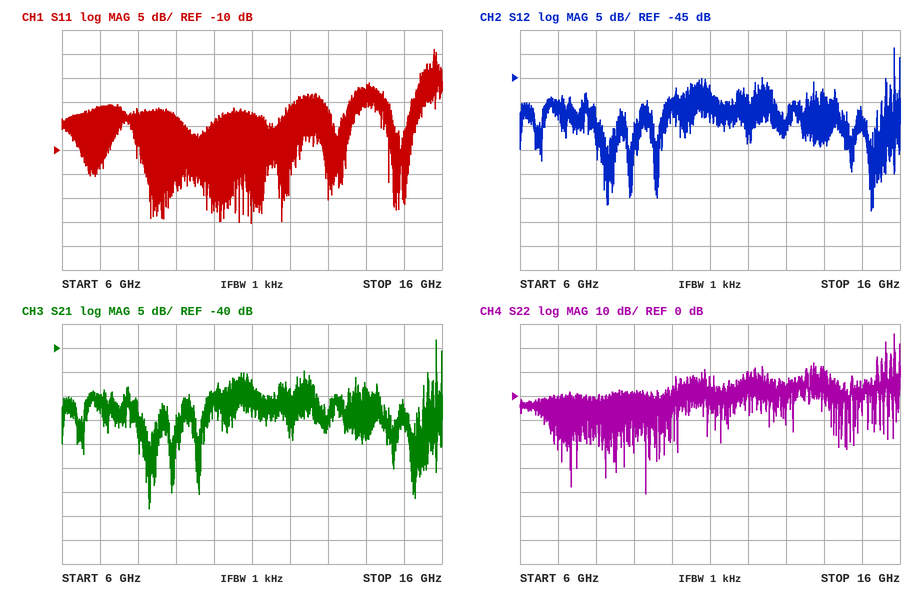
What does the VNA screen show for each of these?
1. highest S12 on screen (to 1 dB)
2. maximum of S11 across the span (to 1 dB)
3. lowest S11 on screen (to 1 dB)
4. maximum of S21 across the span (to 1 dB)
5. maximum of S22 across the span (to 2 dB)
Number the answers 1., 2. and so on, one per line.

1. -39 dB
2. 11 dB
3. -25 dB
4. -38 dB
5. 26 dB
